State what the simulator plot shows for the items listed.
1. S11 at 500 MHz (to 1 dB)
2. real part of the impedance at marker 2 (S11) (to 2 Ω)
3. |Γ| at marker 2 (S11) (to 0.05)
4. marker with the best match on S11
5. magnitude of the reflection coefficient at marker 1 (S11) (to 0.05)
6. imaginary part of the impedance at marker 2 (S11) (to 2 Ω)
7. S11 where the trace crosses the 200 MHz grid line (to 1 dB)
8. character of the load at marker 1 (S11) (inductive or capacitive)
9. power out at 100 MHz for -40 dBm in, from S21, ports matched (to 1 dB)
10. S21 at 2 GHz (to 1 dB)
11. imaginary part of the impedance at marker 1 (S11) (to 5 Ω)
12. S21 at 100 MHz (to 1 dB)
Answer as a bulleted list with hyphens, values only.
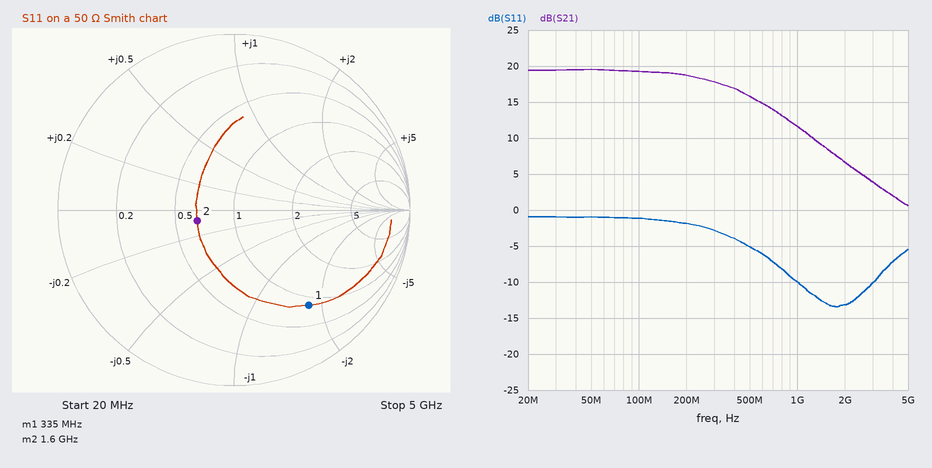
- -5 dB
- 32 Ω
- 0.20
- marker 2
- 0.70
- -4 Ω
- -2 dB
- capacitive
- -21 dBm
- 7 dB
- -85 Ω
- 19 dB
